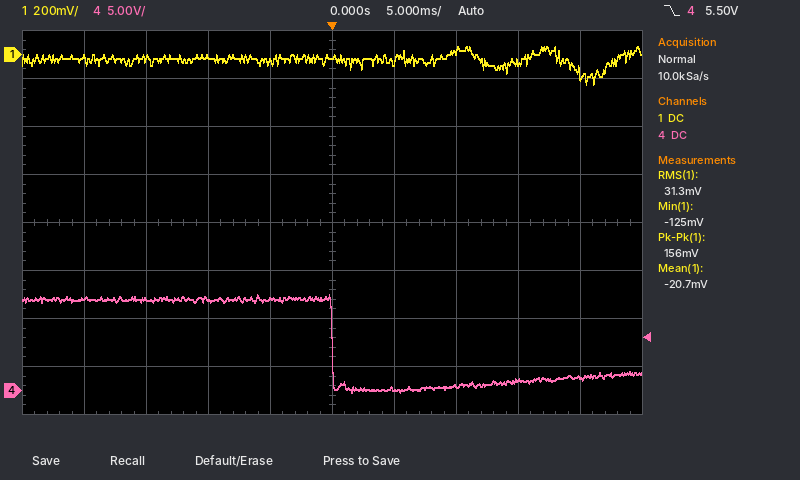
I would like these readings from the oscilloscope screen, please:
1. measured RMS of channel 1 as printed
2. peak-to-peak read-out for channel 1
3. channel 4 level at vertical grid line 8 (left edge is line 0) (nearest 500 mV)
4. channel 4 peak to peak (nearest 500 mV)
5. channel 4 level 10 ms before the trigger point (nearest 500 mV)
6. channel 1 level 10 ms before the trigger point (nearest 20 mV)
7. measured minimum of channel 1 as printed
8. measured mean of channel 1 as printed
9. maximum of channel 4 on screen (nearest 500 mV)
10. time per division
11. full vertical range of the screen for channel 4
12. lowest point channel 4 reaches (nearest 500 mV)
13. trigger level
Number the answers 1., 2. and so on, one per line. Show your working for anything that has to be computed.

1. 31.3 mV
2. 156 mV
3. 1.0 V
4. 10.0 V − (0.0 V) = 10.0 V
5. 9.5 V
6. 0 mV
7. -125 mV
8. -20.7 mV
9. 10.0 V
10. 5 ms
11. 40 V
12. 0.0 V
13. 5.50 V
